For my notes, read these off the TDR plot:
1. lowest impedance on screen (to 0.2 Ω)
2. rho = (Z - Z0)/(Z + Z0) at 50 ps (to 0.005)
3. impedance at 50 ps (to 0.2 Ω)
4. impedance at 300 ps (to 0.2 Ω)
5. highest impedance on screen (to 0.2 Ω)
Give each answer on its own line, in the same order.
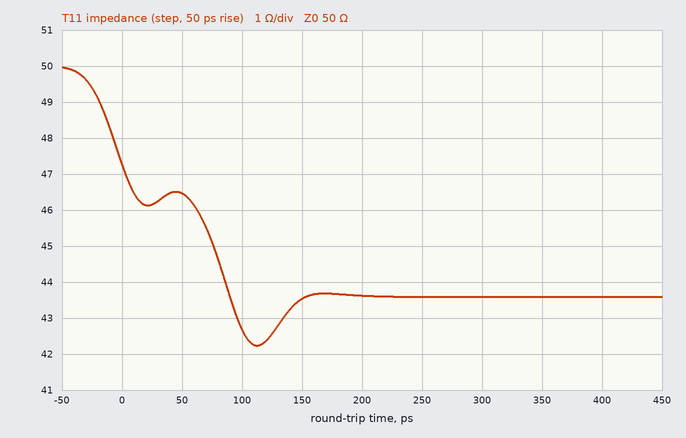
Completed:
42.2 Ω
-0.035
46.4 Ω
43.6 Ω
50.0 Ω
